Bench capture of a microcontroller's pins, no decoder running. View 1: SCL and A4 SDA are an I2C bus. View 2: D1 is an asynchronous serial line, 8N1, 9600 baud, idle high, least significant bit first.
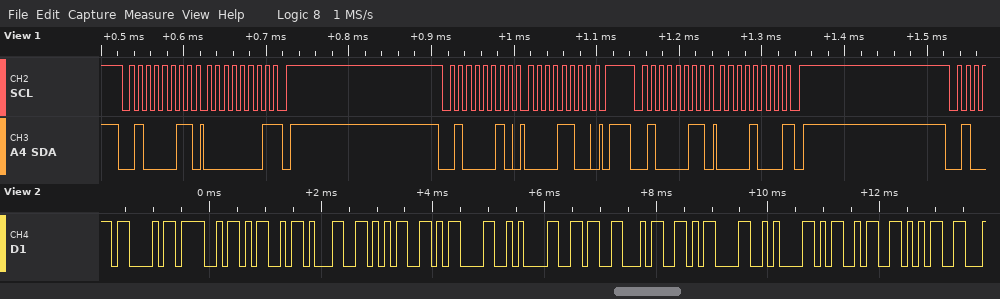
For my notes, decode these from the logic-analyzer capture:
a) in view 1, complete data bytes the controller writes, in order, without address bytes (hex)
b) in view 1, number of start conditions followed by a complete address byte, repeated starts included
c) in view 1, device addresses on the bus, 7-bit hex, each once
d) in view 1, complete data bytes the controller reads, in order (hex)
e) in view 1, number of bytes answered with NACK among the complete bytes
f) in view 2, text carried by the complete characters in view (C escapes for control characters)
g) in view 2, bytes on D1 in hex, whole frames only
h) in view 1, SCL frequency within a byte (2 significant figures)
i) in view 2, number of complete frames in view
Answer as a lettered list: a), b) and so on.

a) 0C
b) 3
c) 0x21
d) 01 08
e) 2
f) "COM15\r\n64\r\nMV"
g) 43 4F 4D 31 35 0D 0A 36 34 0D 0A 4D 56
h) 100 kHz
i) 13
